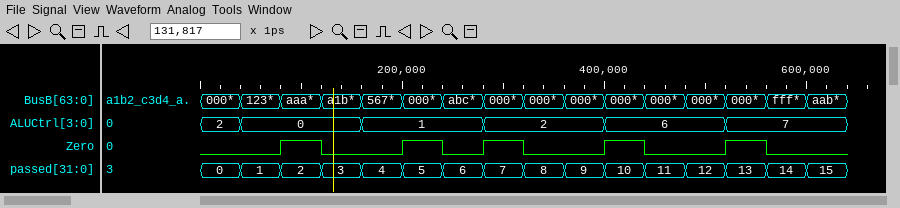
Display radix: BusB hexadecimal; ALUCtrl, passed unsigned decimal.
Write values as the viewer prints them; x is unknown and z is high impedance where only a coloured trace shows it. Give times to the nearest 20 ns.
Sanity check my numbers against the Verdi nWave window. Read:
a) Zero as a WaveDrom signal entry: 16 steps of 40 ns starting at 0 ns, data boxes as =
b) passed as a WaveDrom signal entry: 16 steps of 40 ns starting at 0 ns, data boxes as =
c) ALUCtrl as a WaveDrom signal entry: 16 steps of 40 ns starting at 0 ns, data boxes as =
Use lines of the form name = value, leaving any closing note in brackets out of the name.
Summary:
Zero as a WaveDrom signal entry: 16 steps of 40 ns starting at 0 ns, data boxes as = = {name: 'Zero', wave: '0.10.1010.10.10.'}
passed as a WaveDrom signal entry: 16 steps of 40 ns starting at 0 ns, data boxes as = = {name: 'passed', wave: '================', data: '0 1 2 3 4 5 6 7 8 9 10 11 12 13 14 15'}
ALUCtrl as a WaveDrom signal entry: 16 steps of 40 ns starting at 0 ns, data boxes as = = {name: 'ALUCtrl', wave: '==..=..=..=..=..', data: '2 0 1 2 6 7'}
